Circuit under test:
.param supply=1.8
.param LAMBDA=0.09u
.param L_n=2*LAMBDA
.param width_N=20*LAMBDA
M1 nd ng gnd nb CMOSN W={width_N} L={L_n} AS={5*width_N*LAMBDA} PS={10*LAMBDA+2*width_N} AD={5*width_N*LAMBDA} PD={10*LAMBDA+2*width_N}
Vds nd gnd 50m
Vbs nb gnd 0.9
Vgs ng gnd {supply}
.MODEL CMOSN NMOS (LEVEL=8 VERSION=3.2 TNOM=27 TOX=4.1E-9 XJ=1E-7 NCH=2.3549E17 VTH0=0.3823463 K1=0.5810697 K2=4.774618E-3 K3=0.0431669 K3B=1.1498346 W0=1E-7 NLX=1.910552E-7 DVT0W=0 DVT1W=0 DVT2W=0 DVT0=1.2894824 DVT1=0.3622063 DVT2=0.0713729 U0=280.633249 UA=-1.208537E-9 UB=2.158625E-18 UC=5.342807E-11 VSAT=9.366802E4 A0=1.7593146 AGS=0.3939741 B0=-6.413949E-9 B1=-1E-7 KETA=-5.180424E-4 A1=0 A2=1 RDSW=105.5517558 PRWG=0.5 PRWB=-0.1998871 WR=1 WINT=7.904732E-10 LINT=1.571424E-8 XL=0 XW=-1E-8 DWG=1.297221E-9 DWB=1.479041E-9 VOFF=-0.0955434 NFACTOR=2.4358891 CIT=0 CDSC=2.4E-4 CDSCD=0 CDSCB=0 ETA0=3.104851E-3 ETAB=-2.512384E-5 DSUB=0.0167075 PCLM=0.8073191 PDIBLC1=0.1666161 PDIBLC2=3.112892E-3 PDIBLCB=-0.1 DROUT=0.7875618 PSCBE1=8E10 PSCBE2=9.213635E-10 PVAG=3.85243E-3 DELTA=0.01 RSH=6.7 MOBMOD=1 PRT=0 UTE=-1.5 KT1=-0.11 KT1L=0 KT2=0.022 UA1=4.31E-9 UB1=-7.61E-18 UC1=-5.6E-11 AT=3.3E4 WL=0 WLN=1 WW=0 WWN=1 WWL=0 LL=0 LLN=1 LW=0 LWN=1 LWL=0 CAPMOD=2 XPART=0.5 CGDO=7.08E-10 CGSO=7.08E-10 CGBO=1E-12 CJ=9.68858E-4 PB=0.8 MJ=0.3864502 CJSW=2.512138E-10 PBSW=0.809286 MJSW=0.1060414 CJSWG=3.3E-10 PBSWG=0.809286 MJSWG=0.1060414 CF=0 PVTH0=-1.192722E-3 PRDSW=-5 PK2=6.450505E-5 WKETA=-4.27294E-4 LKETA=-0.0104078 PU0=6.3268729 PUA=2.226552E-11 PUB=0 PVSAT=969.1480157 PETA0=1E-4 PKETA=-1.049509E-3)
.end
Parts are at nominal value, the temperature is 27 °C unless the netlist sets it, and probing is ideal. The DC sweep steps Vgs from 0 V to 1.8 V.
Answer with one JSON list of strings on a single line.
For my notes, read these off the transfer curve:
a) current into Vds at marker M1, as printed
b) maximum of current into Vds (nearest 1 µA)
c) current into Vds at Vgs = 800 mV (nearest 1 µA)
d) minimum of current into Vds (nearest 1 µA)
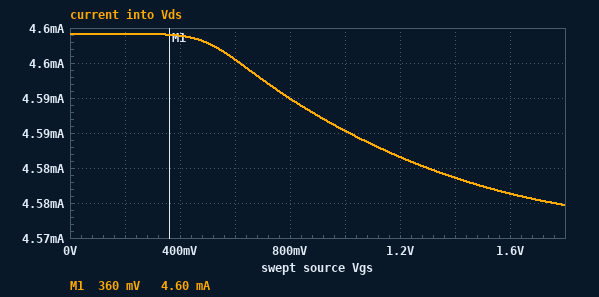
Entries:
["4.60 mA", "4.604 mA", "4.595 mA", "4.580 mA"]
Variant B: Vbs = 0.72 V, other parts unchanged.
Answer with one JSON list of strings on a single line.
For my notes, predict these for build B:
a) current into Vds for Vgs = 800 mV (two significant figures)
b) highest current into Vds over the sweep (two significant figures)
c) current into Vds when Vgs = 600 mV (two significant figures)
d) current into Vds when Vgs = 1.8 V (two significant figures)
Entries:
["-42 µA", "14 µA", "-12 µA", "-120 µA"]
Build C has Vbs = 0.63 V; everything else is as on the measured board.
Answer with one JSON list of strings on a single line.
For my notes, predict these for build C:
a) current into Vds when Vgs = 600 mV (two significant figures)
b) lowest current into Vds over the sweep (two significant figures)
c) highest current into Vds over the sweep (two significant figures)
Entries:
["-25 µA", "-140 µA", "440 nA"]
